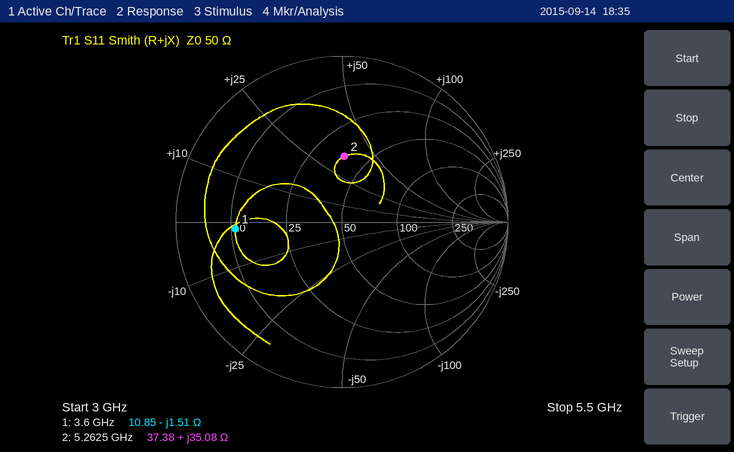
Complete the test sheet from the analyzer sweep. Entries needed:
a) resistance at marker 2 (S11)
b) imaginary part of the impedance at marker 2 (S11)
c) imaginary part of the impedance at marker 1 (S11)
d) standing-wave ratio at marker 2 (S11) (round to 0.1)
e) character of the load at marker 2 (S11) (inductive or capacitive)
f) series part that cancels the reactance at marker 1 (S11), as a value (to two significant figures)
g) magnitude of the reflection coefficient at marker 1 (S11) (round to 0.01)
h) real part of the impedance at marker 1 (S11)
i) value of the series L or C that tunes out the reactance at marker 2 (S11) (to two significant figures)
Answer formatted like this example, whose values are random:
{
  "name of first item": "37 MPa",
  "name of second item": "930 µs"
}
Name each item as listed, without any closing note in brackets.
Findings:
{
  "resistance at marker 2": "37.38 Ω",
  "imaginary part of the impedance at marker 2": "+35.08 Ω",
  "imaginary part of the impedance at marker 1": "-1.51 Ω",
  "standing-wave ratio at marker 2 (S11)": "2.3",
  "character of the load at marker 2 (S11)": "inductive",
  "series part that cancels the reactance at marker 1 (S11), as a value": "67 pH",
  "magnitude of the reflection coefficient at marker 1 (S11)": "0.64",
  "real part of the impedance at marker 1": "10.85 Ω",
  "value of the series L or C that tunes out the reactance at marker 2 (S11)": "860 fF"
}
